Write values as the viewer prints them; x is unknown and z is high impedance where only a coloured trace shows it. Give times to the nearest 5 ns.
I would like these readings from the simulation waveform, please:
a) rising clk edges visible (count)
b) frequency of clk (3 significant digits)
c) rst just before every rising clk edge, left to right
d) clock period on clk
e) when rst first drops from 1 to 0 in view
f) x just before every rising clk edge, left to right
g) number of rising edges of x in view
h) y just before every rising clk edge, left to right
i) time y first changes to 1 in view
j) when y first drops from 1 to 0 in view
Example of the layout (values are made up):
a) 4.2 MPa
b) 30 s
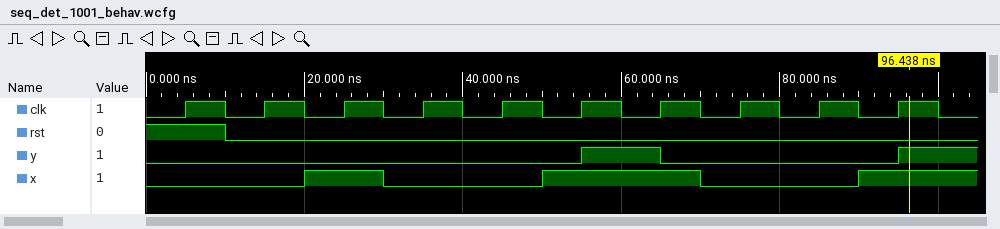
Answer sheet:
a) 10
b) 100 MHz
c) 1 0 0 0 0 0 0 0 0 0
d) 10 ns
e) 10 ns
f) 0 0 1 0 0 1 1 0 0 1
g) 3
h) 0 0 0 0 0 0 1 0 0 0
i) 55 ns
j) 65 ns
